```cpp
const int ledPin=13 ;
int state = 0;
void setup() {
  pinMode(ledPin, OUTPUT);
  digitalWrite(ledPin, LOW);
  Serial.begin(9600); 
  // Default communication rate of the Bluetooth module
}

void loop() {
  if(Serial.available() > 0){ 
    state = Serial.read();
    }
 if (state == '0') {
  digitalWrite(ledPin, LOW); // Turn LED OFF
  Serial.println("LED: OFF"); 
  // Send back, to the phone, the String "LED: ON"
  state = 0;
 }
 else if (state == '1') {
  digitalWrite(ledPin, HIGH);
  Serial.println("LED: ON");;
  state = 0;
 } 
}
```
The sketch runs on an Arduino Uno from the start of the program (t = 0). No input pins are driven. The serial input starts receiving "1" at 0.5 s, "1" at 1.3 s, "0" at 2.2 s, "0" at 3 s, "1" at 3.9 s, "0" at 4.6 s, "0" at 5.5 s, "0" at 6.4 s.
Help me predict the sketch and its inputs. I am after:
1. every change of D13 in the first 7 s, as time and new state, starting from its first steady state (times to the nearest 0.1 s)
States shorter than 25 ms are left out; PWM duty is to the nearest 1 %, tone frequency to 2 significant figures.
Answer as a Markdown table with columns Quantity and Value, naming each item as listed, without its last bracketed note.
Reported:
| Quantity | Value |
|---|---|
| every change of D13 in the first 7 s, as time and new state, starting from its first steady state | 0 s low; 0.5 s high; 2.2 s low; 3.9 s high; 4.6 s low |
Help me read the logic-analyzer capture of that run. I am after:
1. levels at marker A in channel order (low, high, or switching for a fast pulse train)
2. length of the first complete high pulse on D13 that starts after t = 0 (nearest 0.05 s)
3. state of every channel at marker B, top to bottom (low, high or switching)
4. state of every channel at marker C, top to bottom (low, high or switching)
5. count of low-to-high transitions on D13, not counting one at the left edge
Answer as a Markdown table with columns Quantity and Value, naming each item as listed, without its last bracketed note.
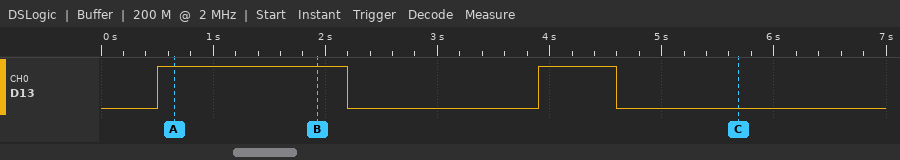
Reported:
| Quantity | Value |
|---|---|
| levels at marker A in channel order | D13 high |
| length of the first complete high pulse on D13 that starts after t = 0 | 1.70 s |
| state of every channel at marker B, top to bottom | D13 high |
| state of every channel at marker C, top to bottom | D13 low |
| count of low-to-high transitions on D13, not counting one at the left edge | 2 |
